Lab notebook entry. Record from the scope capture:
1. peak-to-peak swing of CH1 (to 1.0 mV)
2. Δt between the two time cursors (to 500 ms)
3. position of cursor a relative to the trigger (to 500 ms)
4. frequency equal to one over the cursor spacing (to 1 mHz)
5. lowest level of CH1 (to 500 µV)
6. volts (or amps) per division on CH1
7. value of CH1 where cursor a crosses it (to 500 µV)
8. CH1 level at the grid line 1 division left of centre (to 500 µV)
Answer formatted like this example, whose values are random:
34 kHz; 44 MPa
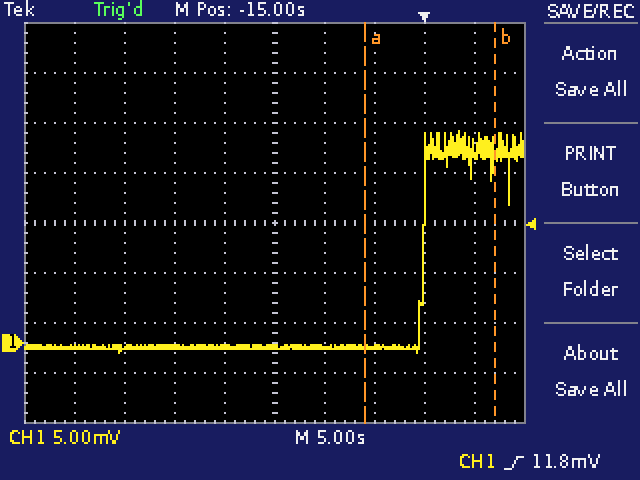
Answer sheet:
22.0 mV; 13.0 s; -6.0 s; 77 mHz; -1.0 mV; 5 mV; -500 µV; -500 µV
